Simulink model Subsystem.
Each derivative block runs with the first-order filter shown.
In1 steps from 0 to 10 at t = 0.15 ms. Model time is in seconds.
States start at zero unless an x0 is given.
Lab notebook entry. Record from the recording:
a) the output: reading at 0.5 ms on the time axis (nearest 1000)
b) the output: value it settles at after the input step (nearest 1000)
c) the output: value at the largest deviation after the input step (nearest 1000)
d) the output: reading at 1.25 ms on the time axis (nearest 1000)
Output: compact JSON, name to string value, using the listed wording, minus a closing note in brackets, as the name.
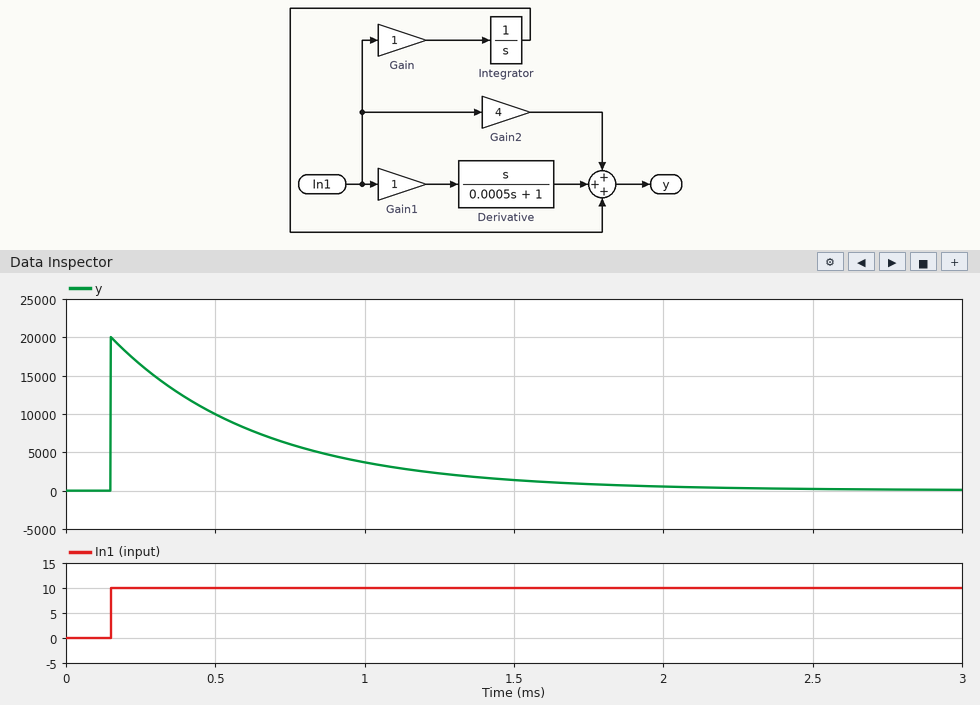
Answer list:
{"the output: reading at 0.5 ms on the time axis": "10000", "the output: value it settles at after the input step": "0", "the output: value at the largest deviation after the input step": "20000", "the output: reading at 1.25 ms on the time axis": "2000"}
